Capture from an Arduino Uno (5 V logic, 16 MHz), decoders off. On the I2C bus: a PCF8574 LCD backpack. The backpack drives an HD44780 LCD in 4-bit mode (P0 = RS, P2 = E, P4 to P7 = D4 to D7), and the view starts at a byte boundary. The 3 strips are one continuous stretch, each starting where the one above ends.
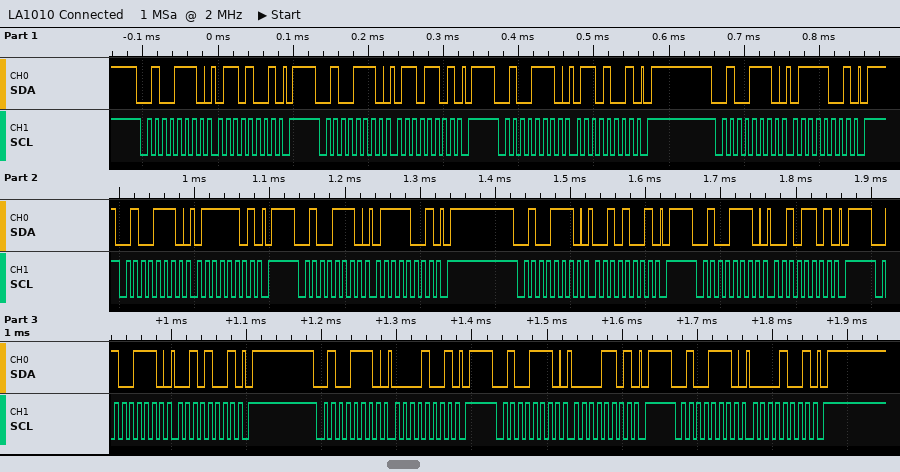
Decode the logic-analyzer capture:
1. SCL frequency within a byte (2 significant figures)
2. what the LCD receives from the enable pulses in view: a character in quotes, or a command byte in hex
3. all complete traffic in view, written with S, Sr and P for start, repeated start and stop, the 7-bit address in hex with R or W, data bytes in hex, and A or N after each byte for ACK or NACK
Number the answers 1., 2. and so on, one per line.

1. 100 kHz
2. 'g' ' '
3. S 27W A 69 A P S 27W A 6D A P S 27W A 69 A P S 27W A 79 A P S 27W A 7D A P S 27W A 79 A P S 27W A 29 A P S 27W A 2D A P S 27W A 29 A P S 27W A 09 A P S 27W A 0D A P S 27W A 09 A P
